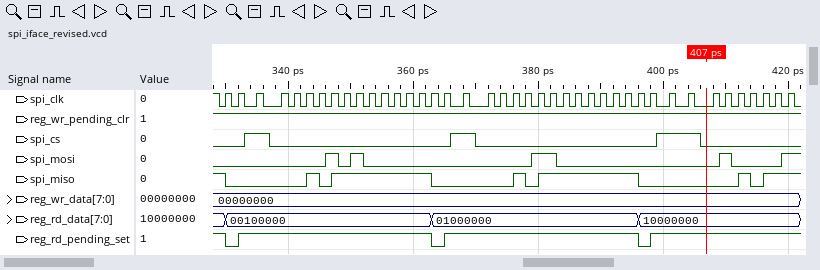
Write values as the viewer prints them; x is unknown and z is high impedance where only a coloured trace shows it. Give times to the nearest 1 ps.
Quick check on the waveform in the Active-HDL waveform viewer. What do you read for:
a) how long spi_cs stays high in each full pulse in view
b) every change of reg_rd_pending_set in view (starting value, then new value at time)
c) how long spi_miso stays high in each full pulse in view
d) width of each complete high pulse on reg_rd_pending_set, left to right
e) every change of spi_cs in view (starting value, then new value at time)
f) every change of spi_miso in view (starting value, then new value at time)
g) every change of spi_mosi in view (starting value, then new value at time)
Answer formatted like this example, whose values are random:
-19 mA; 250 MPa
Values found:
4 ps, 4 ps, 7 ps; 1, 0 at 330 ps, 1 at 332 ps, 0 at 363 ps, 1 at 365 ps, 0 at 396 ps, 1 at 398 ps; 2 ps, 16 ps, 2 ps, 16 ps, 2 ps; 31 ps, 31 ps; 0, 1 at 333 ps, 0 at 337 ps, 1 at 366 ps, 0 at 370 ps, 1 at 399 ps, 0 at 406 ps; 1, 0 at 330 ps, 1 at 343 ps, 0 at 345 ps, 1 at 347 ps, 0 at 363 ps, 1 at 376 ps, 0 at 378 ps, 1 at 380 ps, 0 at 396 ps, 1 at 412 ps, 0 at 414 ps, 1 at 416 ps; 0, 1 at 346 ps, 0 at 348 ps, 1 at 350 ps, 0 at 352 ps, 1 at 379 ps, 0 at 383 ps, 1 at 409 ps, 0 at 411 ps, 1 at 419 ps
